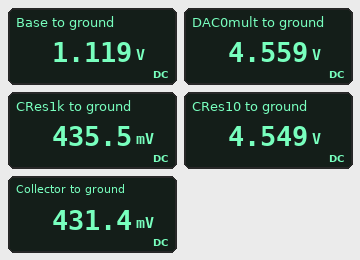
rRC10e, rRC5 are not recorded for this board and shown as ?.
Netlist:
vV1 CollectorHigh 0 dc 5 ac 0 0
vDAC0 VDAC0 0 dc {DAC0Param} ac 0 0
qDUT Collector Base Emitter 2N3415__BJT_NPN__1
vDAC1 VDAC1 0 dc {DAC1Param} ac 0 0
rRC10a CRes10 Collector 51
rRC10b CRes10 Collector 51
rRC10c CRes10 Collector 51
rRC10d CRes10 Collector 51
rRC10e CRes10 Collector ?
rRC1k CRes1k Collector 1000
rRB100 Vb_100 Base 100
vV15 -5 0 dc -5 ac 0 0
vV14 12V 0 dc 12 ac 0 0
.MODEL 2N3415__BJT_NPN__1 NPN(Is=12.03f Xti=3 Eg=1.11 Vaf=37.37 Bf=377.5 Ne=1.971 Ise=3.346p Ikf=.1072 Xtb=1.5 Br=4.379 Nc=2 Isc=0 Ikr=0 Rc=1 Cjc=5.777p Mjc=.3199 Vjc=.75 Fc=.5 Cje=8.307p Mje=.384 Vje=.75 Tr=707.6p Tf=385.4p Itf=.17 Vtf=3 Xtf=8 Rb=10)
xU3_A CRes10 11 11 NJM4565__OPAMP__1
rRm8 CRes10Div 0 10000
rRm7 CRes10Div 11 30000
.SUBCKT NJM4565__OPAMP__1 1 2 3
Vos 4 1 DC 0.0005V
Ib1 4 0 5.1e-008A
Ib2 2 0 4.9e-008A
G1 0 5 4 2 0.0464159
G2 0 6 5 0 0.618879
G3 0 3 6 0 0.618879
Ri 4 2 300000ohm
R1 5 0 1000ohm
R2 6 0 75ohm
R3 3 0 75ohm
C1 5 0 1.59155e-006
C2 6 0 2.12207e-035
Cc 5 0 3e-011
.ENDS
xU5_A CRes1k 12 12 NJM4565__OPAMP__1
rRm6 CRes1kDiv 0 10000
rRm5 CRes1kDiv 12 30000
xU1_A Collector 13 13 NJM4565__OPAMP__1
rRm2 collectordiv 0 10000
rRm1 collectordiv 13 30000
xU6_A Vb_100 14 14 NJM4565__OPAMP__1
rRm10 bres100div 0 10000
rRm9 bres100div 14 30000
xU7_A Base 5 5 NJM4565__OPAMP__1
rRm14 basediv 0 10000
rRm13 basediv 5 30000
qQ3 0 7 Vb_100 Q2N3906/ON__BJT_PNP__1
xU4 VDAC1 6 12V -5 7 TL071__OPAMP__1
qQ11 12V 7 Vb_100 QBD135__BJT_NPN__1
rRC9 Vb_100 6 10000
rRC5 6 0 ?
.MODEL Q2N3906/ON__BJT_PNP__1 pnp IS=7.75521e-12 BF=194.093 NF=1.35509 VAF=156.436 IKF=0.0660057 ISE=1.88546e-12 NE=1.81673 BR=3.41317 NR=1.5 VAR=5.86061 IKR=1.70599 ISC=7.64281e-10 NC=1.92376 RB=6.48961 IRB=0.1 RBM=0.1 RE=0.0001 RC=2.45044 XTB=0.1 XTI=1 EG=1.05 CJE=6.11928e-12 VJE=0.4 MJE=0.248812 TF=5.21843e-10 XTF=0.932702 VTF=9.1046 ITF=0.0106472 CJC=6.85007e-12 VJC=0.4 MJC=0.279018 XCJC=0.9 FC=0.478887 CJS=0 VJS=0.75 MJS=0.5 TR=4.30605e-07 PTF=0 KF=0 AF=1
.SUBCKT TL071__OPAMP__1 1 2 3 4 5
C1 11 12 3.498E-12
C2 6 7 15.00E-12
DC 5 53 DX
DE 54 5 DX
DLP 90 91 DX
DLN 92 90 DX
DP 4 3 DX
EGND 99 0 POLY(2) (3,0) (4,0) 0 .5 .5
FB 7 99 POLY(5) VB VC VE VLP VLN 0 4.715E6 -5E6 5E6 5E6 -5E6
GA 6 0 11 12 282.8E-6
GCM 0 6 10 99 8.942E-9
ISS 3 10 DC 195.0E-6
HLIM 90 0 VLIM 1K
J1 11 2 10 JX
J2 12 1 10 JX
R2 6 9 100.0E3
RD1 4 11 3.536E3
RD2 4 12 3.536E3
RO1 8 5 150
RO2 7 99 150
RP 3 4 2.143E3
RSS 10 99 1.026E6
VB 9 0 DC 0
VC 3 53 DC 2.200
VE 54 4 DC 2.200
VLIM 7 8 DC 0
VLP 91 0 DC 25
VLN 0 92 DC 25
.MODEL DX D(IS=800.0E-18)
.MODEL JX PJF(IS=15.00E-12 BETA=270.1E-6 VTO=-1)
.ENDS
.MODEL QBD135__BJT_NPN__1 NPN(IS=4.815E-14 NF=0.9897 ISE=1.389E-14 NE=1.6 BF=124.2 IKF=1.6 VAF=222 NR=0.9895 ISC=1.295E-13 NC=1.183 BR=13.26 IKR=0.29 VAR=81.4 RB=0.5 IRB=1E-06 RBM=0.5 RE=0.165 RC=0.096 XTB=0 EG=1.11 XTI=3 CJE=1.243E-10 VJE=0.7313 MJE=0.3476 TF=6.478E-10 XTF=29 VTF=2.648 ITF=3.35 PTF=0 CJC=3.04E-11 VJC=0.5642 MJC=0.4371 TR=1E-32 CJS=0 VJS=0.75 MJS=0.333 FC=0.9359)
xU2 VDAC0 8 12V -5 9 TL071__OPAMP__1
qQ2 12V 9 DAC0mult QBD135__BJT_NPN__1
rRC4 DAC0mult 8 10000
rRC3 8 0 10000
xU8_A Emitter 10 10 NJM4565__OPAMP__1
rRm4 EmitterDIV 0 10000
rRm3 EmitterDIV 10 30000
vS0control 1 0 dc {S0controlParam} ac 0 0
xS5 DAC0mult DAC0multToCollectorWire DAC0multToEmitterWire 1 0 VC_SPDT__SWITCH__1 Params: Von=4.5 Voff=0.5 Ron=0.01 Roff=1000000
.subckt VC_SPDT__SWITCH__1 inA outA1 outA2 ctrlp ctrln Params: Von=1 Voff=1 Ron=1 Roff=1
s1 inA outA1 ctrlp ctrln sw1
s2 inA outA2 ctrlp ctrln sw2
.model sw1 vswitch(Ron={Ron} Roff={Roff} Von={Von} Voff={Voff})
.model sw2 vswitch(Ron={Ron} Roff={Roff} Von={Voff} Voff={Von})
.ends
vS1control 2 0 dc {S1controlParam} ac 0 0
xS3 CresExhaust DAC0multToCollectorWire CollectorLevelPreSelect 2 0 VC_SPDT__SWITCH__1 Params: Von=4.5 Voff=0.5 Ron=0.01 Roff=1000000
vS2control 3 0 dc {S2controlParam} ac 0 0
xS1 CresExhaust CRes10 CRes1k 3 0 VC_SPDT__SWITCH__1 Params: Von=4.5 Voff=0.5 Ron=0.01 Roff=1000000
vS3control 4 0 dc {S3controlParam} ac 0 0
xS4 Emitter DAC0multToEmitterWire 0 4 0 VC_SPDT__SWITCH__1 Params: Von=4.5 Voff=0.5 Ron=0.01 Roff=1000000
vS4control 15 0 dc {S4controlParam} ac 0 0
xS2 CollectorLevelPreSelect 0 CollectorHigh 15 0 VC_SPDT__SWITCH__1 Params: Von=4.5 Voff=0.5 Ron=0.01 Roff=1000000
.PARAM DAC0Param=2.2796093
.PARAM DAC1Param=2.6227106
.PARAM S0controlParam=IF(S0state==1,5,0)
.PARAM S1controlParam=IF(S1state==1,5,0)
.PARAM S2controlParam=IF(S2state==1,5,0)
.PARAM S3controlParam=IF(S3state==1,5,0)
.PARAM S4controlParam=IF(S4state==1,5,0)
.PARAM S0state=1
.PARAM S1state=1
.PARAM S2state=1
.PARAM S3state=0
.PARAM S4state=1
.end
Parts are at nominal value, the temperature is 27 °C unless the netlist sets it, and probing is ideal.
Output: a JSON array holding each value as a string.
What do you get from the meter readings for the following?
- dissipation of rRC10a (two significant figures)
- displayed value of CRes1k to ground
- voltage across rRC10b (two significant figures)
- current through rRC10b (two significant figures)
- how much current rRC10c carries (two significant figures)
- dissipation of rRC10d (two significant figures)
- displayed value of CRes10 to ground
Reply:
["330 mW", "435.5 mV", "4.1 V", "81 mA", "81 mA", "330 mW", "4.549 V"]
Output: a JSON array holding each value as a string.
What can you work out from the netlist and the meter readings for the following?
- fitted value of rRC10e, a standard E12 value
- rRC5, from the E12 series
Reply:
["150 Ω", "22 kΩ"]
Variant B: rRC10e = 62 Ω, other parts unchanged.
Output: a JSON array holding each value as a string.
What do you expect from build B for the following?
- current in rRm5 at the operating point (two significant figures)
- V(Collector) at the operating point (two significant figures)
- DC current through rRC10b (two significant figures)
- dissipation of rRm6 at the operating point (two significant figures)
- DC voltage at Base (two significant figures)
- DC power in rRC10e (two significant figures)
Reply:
["12 µA", "470 mV", "80 mA", "1.4 µW", "1.1 V", "270 mW"]
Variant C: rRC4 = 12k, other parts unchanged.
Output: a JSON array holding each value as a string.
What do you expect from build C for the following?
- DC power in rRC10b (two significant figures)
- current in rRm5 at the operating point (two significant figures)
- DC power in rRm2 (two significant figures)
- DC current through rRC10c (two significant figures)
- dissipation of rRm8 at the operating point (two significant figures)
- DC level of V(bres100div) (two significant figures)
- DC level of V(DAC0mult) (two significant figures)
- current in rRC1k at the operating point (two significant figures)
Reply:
["400 mW", "12 µA", "1.4 µW", "89 mA", "160 µW", "950 mV", "5.0 V", "4.5 µA"]
